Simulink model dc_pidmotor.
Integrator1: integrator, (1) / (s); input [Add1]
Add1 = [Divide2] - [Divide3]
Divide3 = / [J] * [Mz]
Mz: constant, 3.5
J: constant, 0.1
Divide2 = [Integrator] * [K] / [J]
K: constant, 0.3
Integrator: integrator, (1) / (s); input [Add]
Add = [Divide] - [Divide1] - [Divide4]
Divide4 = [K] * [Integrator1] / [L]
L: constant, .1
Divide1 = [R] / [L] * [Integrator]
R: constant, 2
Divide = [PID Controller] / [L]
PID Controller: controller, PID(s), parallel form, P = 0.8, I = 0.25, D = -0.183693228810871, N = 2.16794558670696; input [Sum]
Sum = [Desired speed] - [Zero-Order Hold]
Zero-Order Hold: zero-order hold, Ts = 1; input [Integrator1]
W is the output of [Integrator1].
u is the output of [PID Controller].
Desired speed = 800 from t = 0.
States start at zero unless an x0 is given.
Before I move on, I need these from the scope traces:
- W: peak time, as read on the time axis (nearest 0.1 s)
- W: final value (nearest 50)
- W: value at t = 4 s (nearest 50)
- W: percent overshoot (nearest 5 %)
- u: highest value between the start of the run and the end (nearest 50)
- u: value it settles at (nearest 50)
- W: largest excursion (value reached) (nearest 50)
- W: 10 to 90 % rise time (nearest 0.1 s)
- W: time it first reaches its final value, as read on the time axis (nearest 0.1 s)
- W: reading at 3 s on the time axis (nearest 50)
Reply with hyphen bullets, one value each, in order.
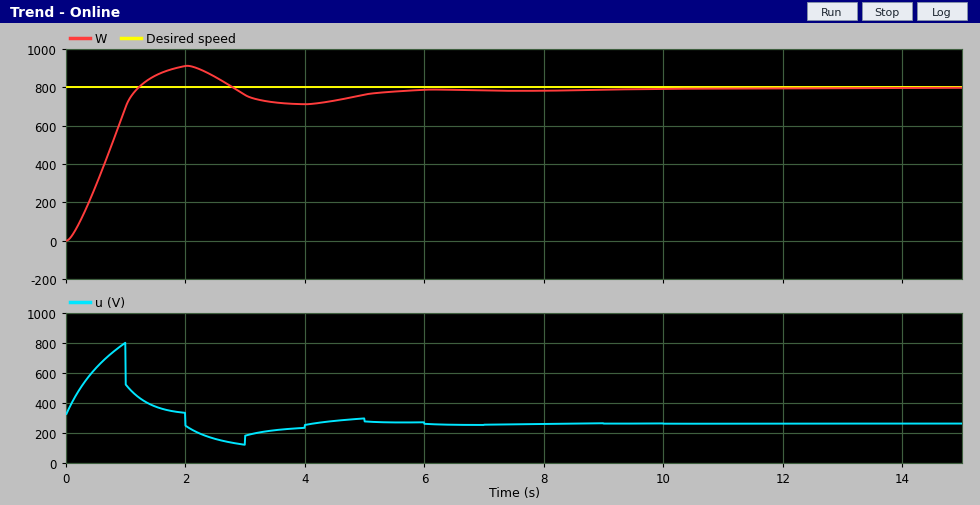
- 2.0 s
- 800
- 700
- 15 %
- 800
- 250
- 900
- 0.8 s
- 1.2 s
- 750
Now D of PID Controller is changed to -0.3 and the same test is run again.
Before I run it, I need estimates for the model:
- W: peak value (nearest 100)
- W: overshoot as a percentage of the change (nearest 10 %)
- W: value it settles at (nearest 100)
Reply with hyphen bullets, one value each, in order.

- 1000
- 30 %
- 800
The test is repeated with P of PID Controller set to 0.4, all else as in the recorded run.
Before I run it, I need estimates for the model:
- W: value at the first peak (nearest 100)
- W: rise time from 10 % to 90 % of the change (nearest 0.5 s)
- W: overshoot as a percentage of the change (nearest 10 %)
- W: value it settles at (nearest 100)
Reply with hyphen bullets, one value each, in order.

- 1000
- 1.5 s
- 20 %
- 800
